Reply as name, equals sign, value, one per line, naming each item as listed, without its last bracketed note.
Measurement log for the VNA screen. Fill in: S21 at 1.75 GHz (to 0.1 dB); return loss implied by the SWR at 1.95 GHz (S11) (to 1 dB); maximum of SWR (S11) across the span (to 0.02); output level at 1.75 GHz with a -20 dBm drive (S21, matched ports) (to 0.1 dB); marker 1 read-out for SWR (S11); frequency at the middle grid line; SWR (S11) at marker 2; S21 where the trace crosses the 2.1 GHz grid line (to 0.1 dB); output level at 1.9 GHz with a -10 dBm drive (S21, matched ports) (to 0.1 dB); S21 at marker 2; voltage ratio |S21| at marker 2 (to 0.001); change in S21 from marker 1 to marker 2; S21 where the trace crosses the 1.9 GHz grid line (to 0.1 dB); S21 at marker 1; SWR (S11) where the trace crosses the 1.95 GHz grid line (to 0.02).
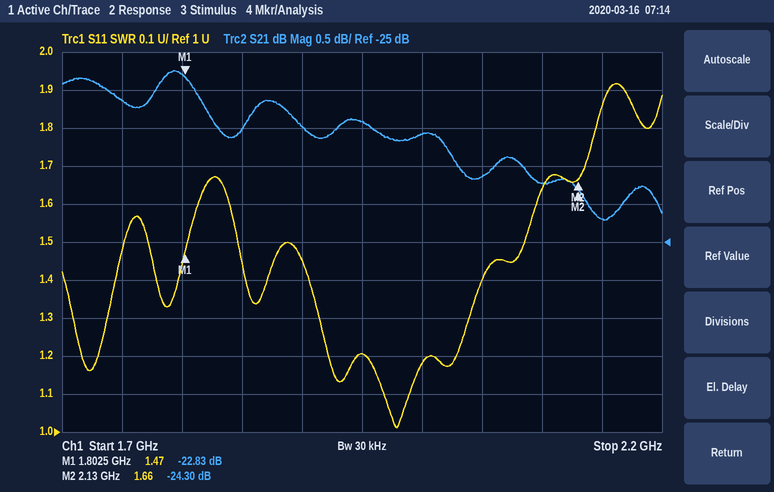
S21 at 1.75 GHz = -23.1 dB
return loss implied by the SWR at 1.95 GHz (S11) = 21 dB
maximum of SWR (S11) across the span = 1.92
output level at 1.75 GHz with a -20 dBm drive (S21, matched ports) = -43.1 dBm
marker 1 read-out for SWR = 1.47
frequency at the middle grid line = 1.95 GHz
SWR (S11) at marker 2 = 1.66
S21 where the trace crosses the 2.1 GHz grid line = -24.2 dB
output level at 1.9 GHz with a -10 dBm drive (S21, matched ports) = -33.5 dBm
S21 at marker 2 = -24.30 dB
voltage ratio |S21| at marker 2 = 0.061
change in S21 from marker 1 to marker 2 = -1.47 dB
S21 where the trace crosses the 1.9 GHz grid line = -23.5 dB
S21 at marker 1 = -22.83 dB
SWR (S11) where the trace crosses the 1.95 GHz grid line = 1.20
